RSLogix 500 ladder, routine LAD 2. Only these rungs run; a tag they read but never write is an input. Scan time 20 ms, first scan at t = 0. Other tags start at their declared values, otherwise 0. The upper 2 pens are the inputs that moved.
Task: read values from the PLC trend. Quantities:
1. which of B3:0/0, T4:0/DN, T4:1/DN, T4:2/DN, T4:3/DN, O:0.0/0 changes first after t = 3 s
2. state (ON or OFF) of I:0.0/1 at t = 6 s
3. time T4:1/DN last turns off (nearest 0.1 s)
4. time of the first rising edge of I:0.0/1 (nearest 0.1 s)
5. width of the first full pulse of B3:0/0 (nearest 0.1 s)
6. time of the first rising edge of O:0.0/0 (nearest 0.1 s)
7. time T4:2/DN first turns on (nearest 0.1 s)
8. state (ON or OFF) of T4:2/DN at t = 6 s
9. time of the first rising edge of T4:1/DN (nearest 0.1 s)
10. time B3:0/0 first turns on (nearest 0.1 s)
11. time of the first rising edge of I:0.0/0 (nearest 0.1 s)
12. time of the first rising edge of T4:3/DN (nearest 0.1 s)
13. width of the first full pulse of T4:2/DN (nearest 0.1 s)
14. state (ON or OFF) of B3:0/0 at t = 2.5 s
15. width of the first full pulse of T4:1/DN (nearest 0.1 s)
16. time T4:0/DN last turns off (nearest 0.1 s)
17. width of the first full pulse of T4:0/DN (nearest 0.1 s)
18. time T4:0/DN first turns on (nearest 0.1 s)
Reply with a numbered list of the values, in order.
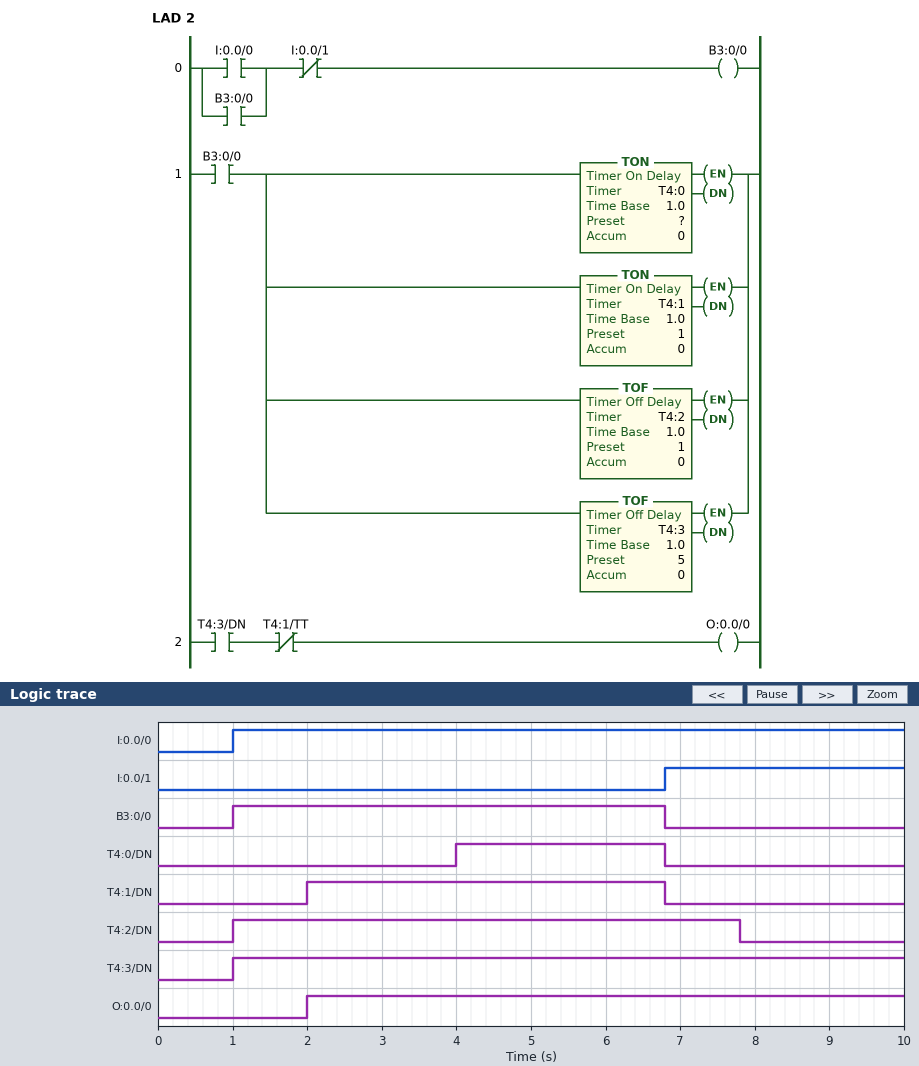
1. T4:0/DN
2. OFF
3. 6.8 s
4. 6.8 s
5. 5.8 s
6. 2.0 s
7. 1.0 s
8. ON
9. 2.0 s
10. 1.0 s
11. 1.0 s
12. 1.0 s
13. 6.8 s
14. ON
15. 4.8 s
16. 6.8 s
17. 2.8 s
18. 4.0 s
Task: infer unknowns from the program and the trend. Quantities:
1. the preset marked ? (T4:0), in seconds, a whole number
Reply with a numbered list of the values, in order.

1. 3 s
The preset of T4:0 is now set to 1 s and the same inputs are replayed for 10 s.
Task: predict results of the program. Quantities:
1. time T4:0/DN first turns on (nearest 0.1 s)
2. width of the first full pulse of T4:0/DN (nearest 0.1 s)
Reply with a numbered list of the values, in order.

1. 2.0 s
2. 4.8 s
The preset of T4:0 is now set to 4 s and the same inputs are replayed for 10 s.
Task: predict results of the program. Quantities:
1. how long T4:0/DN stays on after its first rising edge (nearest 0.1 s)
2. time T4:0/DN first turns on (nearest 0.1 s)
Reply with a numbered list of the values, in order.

1. 1.8 s
2. 5.0 s
